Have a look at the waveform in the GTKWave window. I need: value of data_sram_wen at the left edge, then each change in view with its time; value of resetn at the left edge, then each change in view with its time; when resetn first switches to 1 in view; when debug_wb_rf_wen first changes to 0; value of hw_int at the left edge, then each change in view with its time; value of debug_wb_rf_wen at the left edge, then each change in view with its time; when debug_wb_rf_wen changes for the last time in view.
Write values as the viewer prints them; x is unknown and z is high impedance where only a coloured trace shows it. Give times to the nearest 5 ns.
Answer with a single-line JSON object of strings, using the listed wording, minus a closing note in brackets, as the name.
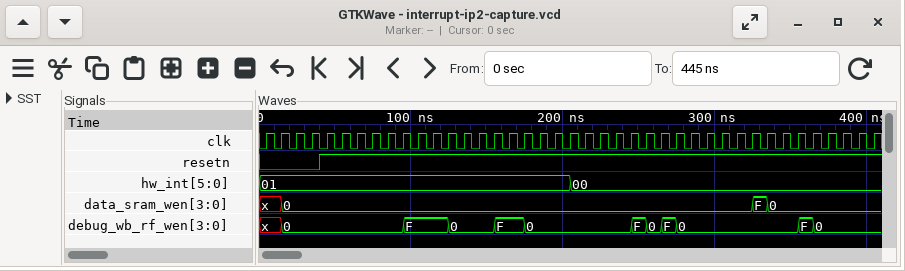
{"value of data_sram_wen at the left edge, then each change in view with its time": "x, 0 at 15 ns, F at 325 ns, 0 at 335 ns", "value of resetn at the left edge, then each change in view with its time": "0, 1 at 40 ns", "when resetn first switches to 1 in view": "40 ns", "when debug_wb_rf_wen first changes to 0": "15 ns", "value of hw_int at the left edge, then each change in view with its time": "01, 00 at 205 ns", "value of debug_wb_rf_wen at the left edge, then each change in view with its time": "x, 0 at 15 ns, F at 95 ns, 0 at 125 ns, F at 155 ns, 0 at 175 ns, F at 245 ns, 0 at 255 ns, F at 265 ns, 0 at 275 ns, F at 355 ns, 0 at 365 ns", "when debug_wb_rf_wen changes for the last time in view": "365 ns"}
